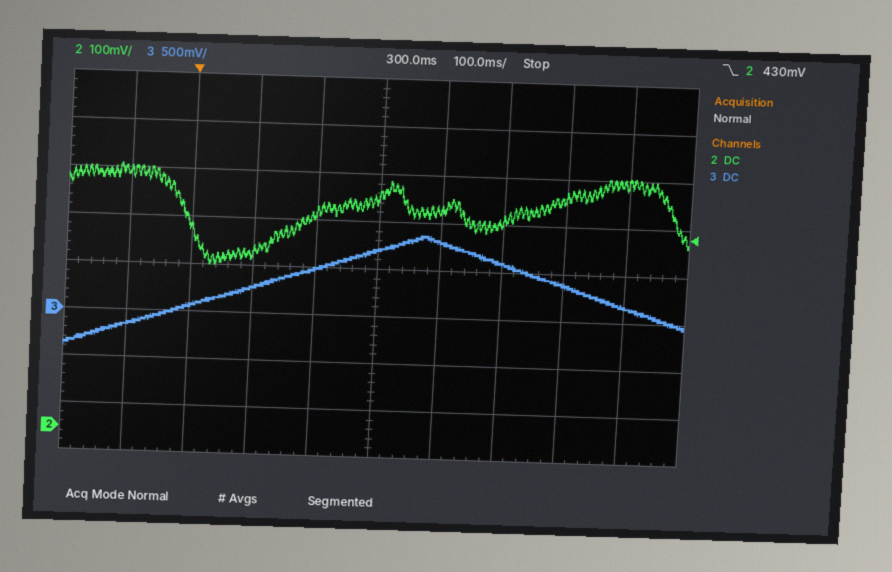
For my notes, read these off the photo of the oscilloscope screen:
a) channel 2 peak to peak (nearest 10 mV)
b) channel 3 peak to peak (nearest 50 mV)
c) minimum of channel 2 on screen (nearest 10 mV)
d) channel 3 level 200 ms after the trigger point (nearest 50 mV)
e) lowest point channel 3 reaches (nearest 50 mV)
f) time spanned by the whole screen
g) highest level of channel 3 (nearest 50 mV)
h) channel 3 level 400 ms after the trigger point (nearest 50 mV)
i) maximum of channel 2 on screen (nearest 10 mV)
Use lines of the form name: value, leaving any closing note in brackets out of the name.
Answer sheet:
channel 2 peak to peak: 210 mV
channel 3 peak to peak: 1.25 V
minimum of channel 2 on screen: 350 mV
channel 3 level 200 ms after the trigger point: 500 mV
lowest point channel 3 reaches: -400 mV
time spanned by the whole screen: 1 s
highest level of channel 3: 850 mV
channel 3 level 400 ms after the trigger point: 800 mV
maximum of channel 2 on screen: 560 mV
